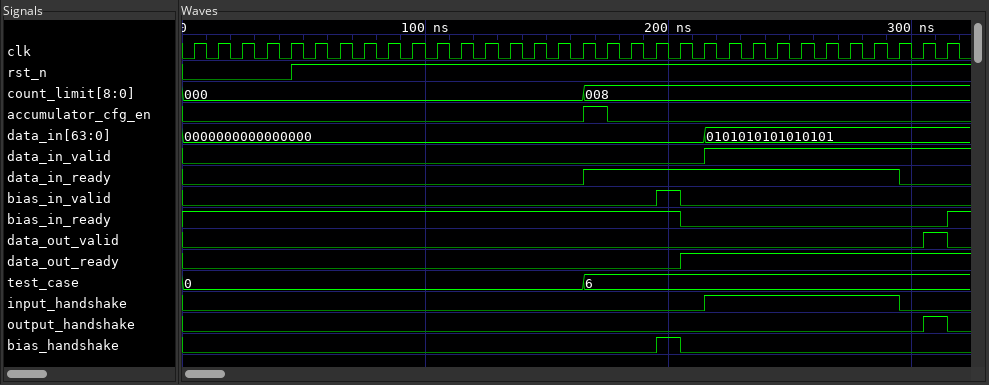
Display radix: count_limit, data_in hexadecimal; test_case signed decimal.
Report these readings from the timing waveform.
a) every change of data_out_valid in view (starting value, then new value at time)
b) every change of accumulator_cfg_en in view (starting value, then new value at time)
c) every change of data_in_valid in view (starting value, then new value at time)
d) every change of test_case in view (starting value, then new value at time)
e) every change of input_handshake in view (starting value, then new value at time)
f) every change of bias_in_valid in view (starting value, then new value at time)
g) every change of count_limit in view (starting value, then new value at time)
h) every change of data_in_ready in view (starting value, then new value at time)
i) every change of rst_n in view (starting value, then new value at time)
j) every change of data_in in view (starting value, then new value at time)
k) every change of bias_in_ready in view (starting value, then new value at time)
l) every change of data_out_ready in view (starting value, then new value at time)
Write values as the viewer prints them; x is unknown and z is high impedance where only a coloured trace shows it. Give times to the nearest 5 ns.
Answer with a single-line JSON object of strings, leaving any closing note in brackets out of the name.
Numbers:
{"every change of data_out_valid in view": "0, 1 at 305 ns, 0 at 315 ns", "every change of accumulator_cfg_en in view": "0, 1 at 165 ns, 0 at 175 ns", "every change of data_in_valid in view": "0, 1 at 215 ns", "every change of test_case in view": "0, 6 at 165 ns", "every change of input_handshake in view": "0, 1 at 215 ns, 0 at 295 ns", "every change of bias_in_valid in view": "0, 1 at 195 ns, 0 at 205 ns", "every change of count_limit in view": "000, 008 at 165 ns", "every change of data_in_ready in view": "0, 1 at 165 ns, 0 at 295 ns", "every change of rst_n in view": "0, 1 at 45 ns", "every change of data_in in view": "0000000000000000, 0101010101010101 at 215 ns", "every change of bias_in_ready in view": "1, 0 at 205 ns, 1 at 315 ns", "every change of data_out_ready in view": "0, 1 at 205 ns"}
